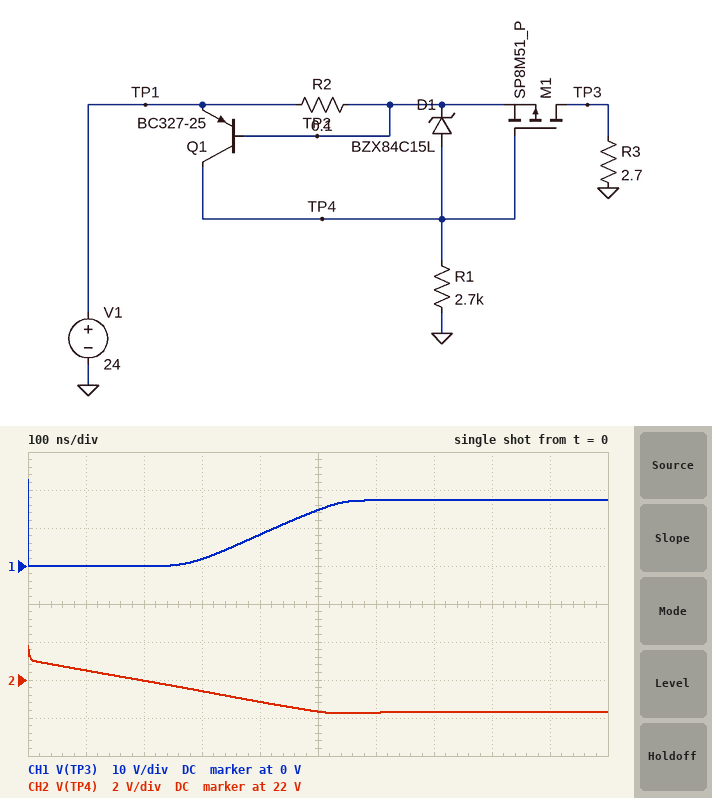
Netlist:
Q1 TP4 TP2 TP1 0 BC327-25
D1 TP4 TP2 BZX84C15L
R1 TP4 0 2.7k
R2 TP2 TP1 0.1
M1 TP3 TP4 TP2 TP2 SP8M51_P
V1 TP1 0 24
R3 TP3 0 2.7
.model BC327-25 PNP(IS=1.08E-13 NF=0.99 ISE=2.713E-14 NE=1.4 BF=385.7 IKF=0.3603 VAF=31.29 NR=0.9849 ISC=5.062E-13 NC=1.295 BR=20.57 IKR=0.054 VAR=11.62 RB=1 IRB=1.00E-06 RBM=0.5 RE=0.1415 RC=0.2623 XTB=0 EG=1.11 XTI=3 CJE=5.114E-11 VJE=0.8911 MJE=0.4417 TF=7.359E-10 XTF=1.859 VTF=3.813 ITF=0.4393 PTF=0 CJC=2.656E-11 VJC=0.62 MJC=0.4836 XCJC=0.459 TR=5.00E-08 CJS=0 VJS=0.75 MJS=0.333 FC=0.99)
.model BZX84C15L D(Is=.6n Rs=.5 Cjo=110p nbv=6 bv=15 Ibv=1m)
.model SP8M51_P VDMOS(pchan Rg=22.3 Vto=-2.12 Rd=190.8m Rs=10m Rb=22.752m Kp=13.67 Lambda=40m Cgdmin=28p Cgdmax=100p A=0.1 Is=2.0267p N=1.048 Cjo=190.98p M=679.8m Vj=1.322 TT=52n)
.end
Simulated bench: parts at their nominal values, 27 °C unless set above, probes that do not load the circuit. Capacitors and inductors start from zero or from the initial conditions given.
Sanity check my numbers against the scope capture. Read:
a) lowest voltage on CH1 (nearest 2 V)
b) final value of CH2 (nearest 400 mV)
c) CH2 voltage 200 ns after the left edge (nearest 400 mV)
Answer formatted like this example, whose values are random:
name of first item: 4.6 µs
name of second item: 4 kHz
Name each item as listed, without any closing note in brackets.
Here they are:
lowest voltage on CH1: 0 V
final value of CH2: 20.4 V
CH2 voltage 200 ns after the left edge: 22.0 V
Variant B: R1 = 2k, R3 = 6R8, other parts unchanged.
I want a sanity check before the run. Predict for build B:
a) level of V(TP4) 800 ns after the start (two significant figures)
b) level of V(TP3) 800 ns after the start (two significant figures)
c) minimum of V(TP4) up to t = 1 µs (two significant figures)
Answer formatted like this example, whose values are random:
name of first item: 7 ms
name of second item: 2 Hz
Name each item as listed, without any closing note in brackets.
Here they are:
level of V(TP4) 800 ns after the start: 18 V
level of V(TP3) 800 ns after the start: 23 V
minimum of V(TP4) up to t = 1 µs: 17 V
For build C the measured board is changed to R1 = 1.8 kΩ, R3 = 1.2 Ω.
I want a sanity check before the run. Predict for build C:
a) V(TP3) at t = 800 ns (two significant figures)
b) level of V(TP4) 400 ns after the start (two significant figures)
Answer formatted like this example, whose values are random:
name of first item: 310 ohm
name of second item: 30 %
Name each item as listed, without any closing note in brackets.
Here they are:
V(TP3) at t = 800 ns: 7.8 V
level of V(TP4) 400 ns after the start: 20 V
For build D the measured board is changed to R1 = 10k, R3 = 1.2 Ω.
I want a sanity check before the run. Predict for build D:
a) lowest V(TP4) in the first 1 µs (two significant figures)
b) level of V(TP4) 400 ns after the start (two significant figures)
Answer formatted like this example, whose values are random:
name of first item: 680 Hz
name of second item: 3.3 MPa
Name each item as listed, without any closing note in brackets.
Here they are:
lowest V(TP4) in the first 1 µs: 22 V
level of V(TP4) 400 ns after the start: 23 V
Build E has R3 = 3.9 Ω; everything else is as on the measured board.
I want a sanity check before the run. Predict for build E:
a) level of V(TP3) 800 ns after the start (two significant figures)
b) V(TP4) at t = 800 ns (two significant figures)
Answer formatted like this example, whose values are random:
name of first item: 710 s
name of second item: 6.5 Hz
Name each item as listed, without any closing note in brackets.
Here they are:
level of V(TP3) 800 ns after the start: 22 V
V(TP4) at t = 800 ns: 19 V
